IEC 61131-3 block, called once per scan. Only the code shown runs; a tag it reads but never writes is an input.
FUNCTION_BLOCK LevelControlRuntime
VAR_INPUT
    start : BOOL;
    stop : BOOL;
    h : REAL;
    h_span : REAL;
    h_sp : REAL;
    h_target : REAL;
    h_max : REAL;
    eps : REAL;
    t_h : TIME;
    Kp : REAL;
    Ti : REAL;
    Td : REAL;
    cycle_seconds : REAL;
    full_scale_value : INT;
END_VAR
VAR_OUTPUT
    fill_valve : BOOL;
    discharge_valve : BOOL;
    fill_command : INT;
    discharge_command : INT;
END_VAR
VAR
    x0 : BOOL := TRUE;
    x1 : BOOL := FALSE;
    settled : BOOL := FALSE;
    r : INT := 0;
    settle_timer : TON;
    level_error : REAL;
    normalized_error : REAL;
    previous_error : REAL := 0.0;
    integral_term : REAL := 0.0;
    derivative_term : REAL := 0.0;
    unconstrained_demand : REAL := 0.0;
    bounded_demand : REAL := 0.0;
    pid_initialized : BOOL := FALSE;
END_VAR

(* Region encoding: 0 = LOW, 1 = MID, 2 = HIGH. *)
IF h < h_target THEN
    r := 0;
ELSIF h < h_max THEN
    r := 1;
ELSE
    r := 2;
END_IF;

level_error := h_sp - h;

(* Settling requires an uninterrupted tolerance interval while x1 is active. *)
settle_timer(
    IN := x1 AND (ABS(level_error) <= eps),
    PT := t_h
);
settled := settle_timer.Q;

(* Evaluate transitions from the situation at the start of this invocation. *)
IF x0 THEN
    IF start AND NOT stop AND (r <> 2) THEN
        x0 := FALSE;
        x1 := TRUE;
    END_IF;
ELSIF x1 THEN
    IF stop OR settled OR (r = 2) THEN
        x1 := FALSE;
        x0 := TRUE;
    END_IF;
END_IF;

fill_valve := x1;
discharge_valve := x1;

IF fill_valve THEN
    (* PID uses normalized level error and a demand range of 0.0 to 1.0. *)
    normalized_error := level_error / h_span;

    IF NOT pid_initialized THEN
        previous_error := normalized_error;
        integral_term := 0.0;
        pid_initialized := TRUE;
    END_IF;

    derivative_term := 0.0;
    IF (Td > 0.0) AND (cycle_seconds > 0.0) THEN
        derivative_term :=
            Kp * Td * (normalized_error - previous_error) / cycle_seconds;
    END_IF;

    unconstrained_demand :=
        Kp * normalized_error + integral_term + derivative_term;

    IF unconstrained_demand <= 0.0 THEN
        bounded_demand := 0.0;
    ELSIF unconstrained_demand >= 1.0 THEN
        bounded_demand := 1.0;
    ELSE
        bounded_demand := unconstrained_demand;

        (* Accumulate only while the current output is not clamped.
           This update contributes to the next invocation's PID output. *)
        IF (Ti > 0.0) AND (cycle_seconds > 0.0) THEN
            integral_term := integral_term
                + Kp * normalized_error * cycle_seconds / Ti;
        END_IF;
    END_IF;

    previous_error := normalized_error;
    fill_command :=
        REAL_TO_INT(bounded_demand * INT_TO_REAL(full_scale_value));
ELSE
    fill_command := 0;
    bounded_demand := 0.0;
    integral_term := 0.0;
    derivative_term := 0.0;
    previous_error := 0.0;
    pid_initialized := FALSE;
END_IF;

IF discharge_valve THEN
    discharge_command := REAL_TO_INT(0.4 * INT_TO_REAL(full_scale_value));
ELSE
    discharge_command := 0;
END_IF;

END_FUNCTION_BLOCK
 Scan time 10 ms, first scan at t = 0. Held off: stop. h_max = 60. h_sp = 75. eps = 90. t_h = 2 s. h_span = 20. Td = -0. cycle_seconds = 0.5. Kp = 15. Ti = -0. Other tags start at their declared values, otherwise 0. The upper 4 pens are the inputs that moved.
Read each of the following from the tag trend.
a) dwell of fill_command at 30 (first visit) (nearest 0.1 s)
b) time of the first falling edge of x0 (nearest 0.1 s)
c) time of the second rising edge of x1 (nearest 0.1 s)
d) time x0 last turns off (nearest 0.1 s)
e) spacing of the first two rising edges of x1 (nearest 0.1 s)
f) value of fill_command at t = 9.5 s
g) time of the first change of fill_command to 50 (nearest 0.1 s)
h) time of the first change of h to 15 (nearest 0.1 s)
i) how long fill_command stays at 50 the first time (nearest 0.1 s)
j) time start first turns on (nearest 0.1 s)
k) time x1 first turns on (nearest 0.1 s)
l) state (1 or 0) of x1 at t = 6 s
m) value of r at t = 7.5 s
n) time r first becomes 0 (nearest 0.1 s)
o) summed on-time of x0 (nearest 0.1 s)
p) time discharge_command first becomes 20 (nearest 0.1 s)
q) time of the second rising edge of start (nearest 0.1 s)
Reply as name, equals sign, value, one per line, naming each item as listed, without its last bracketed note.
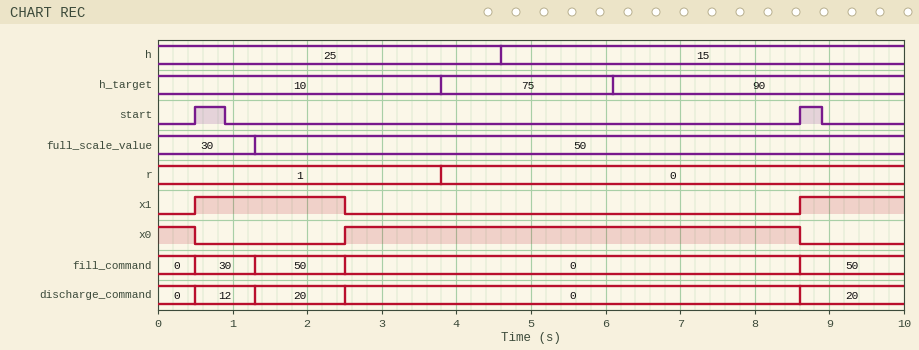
dwell of fill_command at 30 (first visit) = 0.8 s
time of the first falling edge of x0 = 0.5 s
time of the second rising edge of x1 = 8.6 s
time x0 last turns off = 8.6 s
spacing of the first two rising edges of x1 = 8.1 s
value of fill_command at t = 9.5 s = 50
time of the first change of fill_command to 50 = 1.3 s
time of the first change of h to 15 = 4.6 s
how long fill_command stays at 50 the first time = 1.2 s
time start first turns on = 0.5 s
time x1 first turns on = 0.5 s
state (1 or 0) of x1 at t = 6 s = 0
value of r at t = 7.5 s = 0
time r first becomes 0 = 3.8 s
summed on-time of x0 = 6.6 s
time discharge_command first becomes 20 = 1.3 s
time of the second rising edge of start = 8.6 s
